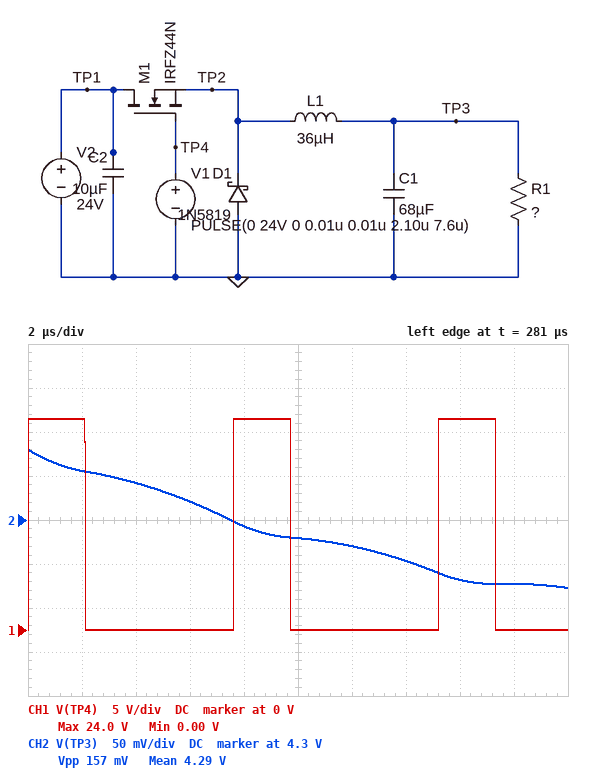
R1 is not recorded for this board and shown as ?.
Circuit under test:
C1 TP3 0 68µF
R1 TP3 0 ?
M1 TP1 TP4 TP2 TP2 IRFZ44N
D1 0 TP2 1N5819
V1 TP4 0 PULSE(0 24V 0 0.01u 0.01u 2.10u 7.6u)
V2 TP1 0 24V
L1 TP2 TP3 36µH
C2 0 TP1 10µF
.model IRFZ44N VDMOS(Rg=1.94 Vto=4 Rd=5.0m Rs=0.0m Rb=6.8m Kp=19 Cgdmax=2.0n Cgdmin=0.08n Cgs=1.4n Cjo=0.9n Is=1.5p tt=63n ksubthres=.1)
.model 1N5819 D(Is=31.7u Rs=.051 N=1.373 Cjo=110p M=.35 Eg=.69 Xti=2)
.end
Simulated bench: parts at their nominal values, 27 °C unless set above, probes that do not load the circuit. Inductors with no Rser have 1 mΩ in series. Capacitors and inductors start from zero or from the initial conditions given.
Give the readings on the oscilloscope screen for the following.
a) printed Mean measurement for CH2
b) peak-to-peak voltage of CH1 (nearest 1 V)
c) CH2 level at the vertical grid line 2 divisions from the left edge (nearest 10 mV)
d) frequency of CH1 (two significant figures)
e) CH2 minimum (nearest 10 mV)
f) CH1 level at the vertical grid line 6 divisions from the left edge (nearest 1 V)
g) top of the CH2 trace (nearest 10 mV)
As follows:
4.29 V
24 V
4.34 V
130 kHz
4.22 V
0 V
4.38 V
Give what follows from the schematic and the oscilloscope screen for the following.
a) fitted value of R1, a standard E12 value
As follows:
1.5 Ω
